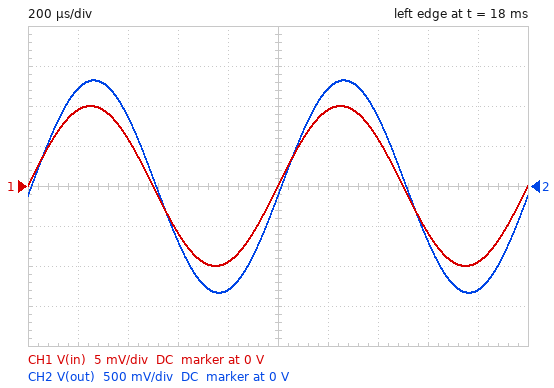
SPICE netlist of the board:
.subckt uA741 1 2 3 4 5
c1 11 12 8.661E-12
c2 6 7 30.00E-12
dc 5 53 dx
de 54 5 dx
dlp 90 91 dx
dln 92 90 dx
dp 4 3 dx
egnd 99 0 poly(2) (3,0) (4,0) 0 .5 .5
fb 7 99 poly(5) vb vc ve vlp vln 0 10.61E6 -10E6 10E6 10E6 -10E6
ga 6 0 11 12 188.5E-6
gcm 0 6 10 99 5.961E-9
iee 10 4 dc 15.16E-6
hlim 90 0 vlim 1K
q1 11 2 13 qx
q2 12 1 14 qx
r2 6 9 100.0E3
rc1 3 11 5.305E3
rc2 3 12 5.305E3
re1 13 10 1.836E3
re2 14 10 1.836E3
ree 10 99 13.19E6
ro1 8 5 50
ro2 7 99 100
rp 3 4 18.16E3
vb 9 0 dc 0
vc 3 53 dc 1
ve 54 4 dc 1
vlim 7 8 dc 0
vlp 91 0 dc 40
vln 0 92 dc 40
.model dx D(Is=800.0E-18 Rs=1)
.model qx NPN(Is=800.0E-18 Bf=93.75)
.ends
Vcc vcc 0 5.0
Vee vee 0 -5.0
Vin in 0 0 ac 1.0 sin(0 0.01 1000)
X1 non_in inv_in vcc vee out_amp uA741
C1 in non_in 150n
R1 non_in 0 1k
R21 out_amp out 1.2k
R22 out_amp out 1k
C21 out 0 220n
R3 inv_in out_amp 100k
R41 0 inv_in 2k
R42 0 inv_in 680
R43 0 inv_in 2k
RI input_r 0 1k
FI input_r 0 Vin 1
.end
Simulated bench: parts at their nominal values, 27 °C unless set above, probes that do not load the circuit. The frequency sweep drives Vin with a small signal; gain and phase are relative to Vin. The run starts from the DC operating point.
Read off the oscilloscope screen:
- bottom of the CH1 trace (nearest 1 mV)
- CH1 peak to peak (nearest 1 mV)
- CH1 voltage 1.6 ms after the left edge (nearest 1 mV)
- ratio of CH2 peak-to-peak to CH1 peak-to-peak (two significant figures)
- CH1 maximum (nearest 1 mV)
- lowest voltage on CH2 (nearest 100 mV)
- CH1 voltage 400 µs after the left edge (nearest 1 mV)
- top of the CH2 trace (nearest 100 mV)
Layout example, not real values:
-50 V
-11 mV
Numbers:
-10 mV
20 mV
-6 mV
130
10 mV
-1.3 V
6 mV
1.3 V
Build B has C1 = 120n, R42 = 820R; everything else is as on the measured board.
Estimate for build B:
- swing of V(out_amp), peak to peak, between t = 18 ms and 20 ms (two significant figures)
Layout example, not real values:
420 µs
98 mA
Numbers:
2.6 V
